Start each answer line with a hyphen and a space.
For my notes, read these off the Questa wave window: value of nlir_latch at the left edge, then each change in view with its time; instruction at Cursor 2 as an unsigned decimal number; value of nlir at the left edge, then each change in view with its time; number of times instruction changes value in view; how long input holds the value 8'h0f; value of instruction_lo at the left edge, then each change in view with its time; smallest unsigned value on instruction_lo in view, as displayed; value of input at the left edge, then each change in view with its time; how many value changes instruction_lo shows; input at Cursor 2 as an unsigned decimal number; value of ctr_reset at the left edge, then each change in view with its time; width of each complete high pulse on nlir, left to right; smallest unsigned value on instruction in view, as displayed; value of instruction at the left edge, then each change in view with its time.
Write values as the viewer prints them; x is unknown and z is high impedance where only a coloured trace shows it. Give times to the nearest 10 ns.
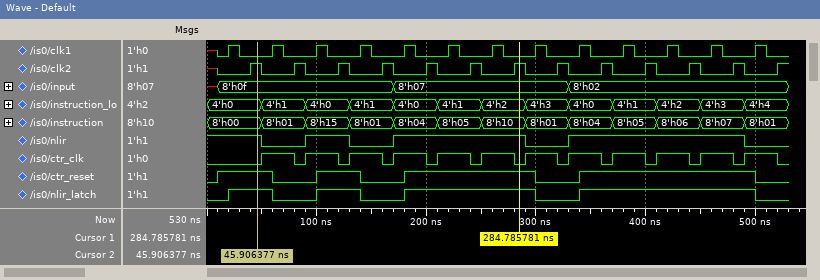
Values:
- 0, 1 at 20 ns, 0 at 60 ns, 1 at 100 ns, 0 at 140 ns, 1 at 180 ns, 0 at 300 ns, 1 at 340 ns, 0 at 500 ns
- 0
- 1, 0 at 50 ns, 1 at 90 ns, 0 at 130 ns, 1 at 170 ns, 0 at 290 ns, 1 at 330 ns, 0 at 490 ns
- 12
- 160 ns
- 4'h0, 4'h1 at 50 ns, 4'h0 at 90 ns, 4'h1 at 130 ns, 4'h0 at 170 ns, 4'h1 at 210 ns, 4'h2 at 250 ns, 4'h3 at 290 ns, 4'h0 at 330 ns, 4'h1 at 370 ns, 4'h2 at 410 ns, 4'h3 at 450 ns, 4'h4 at 490 ns
- 4'h0
- x, 8'h0f at 10 ns, 8'h07 at 170 ns, 8'h02 at 330 ns
- 12
- 15
- 0, 1 at 10 ns, 0 at 60 ns, 1 at 100 ns, 0 at 140 ns, 1 at 180 ns, 0 at 300 ns, 1 at 340 ns, 0 at 500 ns
- 40 ns, 120 ns, 160 ns
- 8'h00
- 8'h00, 8'h01 at 50 ns, 8'h15 at 90 ns, 8'h01 at 130 ns, 8'h04 at 170 ns, 8'h05 at 210 ns, 8'h10 at 250 ns, 8'h01 at 290 ns, 8'h04 at 330 ns, 8'h05 at 370 ns, 8'h06 at 410 ns, 8'h07 at 450 ns, 8'h01 at 490 ns
